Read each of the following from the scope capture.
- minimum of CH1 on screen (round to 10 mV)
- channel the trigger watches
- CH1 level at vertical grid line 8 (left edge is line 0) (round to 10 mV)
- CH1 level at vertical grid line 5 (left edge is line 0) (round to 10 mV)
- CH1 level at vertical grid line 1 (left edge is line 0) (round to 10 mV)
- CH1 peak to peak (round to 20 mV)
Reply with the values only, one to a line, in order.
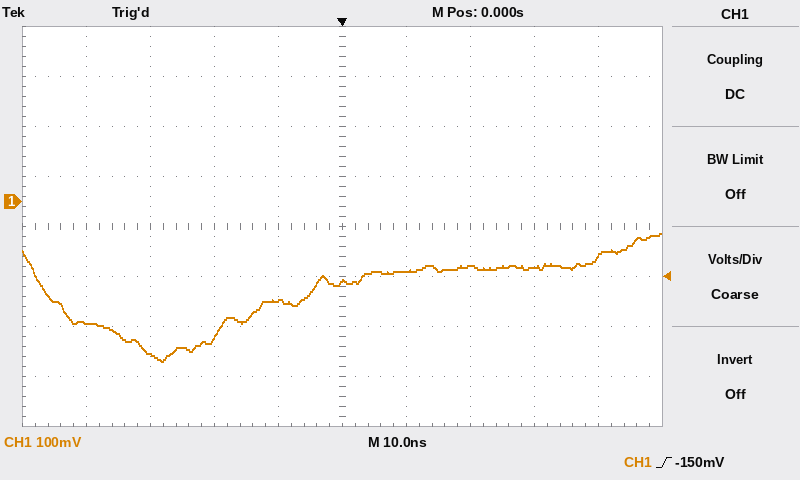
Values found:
-320 mV
CH1
-130 mV
-160 mV
-240 mV
260 mV
